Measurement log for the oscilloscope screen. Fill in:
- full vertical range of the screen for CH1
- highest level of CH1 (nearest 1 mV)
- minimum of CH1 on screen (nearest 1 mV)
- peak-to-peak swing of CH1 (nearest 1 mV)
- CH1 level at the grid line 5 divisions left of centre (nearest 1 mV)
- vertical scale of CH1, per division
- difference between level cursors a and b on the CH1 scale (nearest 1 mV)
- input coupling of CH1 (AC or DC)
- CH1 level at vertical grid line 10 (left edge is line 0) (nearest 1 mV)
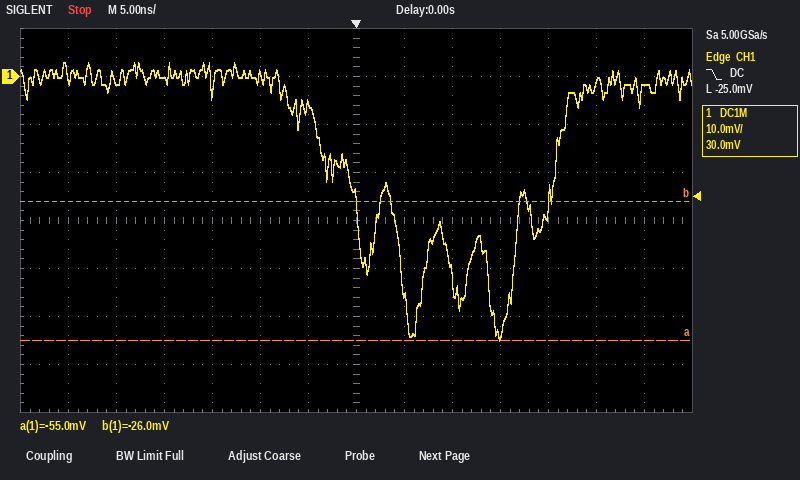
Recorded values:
80 mV
3 mV
-55 mV
58 mV
-1 mV
10 mV
29 mV
DC
-54 mV
